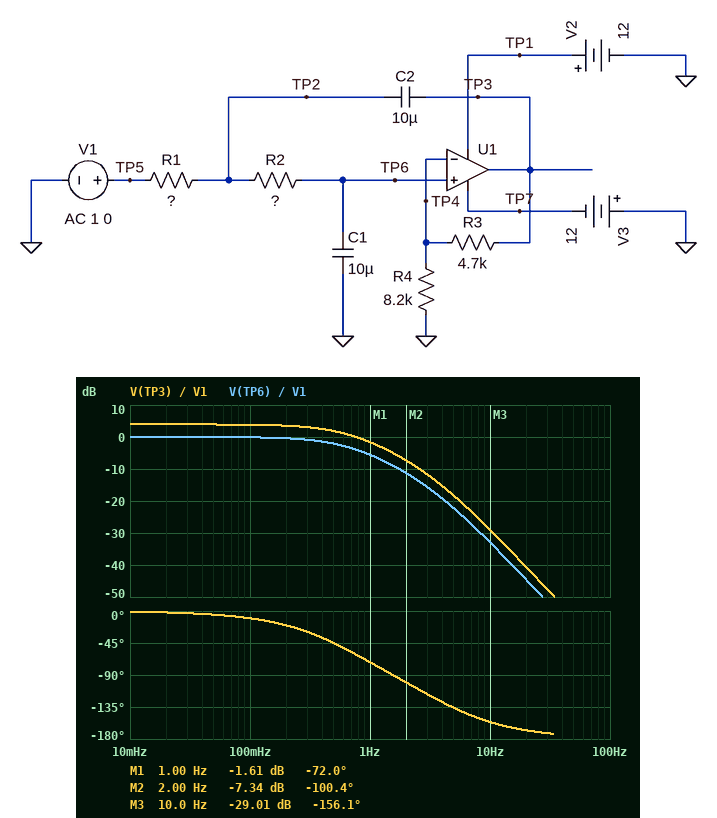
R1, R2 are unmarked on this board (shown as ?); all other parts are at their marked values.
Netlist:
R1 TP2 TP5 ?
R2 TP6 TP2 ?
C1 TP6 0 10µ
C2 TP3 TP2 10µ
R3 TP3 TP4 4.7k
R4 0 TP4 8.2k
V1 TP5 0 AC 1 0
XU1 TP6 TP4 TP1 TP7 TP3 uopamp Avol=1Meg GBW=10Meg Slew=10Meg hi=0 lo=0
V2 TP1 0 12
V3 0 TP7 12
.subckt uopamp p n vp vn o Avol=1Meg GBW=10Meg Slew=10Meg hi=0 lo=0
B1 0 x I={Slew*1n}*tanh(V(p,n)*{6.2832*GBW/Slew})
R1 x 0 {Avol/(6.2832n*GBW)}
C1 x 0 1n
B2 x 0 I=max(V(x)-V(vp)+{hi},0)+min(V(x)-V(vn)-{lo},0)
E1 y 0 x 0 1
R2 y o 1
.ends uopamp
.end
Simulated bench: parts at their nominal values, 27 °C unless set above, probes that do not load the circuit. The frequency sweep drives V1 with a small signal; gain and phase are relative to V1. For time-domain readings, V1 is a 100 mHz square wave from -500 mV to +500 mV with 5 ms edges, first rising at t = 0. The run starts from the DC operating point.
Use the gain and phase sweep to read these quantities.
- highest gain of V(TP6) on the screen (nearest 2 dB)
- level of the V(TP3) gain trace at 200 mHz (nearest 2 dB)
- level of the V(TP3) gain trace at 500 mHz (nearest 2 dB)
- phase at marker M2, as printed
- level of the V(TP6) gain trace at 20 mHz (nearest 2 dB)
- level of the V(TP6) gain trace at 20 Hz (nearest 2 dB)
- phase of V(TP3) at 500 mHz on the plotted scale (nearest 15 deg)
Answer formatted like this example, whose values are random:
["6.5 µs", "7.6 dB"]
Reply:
["0 dB", "4 dB", "2 dB", "-100.4 deg", "0 dB", "-44 dB", "-45 deg"]
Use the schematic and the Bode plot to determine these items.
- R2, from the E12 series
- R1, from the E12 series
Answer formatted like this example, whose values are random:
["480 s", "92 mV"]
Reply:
["27 kΩ", "3.9 kΩ"]
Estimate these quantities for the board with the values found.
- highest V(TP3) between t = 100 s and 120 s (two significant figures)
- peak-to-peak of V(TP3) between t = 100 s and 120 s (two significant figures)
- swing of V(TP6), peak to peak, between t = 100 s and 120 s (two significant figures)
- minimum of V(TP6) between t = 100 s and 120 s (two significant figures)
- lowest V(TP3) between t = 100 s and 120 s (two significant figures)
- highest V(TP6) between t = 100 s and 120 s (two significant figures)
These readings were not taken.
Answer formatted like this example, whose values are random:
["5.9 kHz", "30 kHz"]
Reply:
["790 mV", "1.6 V", "1.0 V", "-500 mV", "-790 mV", "500 mV"]
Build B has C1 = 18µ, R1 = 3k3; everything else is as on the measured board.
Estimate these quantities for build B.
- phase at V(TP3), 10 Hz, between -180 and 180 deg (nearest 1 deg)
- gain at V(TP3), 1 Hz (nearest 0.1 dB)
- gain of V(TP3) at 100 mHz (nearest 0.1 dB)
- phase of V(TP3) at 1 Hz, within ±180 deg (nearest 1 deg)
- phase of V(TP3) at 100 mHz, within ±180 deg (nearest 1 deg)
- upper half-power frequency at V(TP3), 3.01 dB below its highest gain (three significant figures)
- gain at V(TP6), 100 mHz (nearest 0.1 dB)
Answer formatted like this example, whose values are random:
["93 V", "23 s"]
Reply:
["-152 deg", "-6.5 dB", "3.5 dB", "-84 deg", "-18 deg", "321 mHz", "-0.4 dB"]
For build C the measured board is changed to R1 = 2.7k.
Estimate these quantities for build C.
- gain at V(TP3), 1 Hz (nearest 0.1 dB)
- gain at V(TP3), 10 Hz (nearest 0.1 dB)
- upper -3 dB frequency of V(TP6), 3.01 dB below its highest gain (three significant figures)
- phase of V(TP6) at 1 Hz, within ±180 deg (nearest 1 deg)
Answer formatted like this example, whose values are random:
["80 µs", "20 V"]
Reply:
["-1.7 dB", "-26.4 dB", "622 mHz", "-68 deg"]
